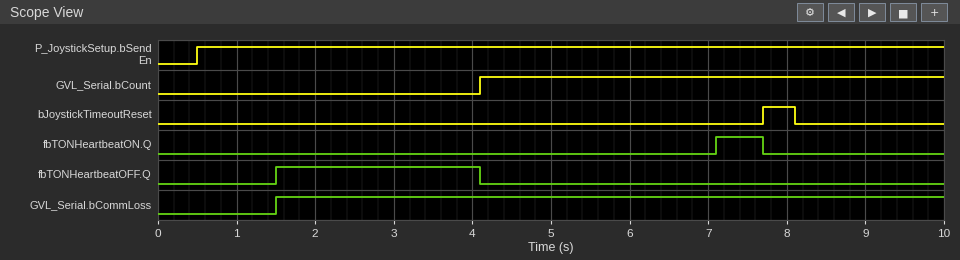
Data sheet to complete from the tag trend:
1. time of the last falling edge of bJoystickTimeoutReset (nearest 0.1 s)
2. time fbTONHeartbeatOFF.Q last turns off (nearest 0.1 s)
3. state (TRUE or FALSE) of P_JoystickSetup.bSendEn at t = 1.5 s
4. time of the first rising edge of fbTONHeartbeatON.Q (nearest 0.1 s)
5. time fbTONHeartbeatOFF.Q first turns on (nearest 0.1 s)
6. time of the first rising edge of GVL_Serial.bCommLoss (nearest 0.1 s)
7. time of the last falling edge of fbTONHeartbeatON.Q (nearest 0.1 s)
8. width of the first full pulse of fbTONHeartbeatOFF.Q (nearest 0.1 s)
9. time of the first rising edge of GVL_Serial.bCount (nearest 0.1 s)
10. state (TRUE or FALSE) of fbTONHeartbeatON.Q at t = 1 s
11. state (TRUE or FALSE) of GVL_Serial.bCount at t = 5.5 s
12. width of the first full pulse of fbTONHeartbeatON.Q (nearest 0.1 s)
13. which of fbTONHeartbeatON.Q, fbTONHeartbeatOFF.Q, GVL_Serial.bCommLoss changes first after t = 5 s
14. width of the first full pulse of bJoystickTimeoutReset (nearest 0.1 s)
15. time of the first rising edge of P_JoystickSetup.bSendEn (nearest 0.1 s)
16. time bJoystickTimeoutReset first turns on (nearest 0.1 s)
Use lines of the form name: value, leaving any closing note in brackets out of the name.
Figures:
time of the last falling edge of bJoystickTimeoutReset: 8.1 s
time fbTONHeartbeatOFF.Q last turns off: 4.1 s
state (TRUE or FALSE) of P_JoystickSetup.bSendEn at t = 1.5 s: TRUE
time of the first rising edge of fbTONHeartbeatON.Q: 7.1 s
time fbTONHeartbeatOFF.Q first turns on: 1.5 s
time of the first rising edge of GVL_Serial.bCommLoss: 1.5 s
time of the last falling edge of fbTONHeartbeatON.Q: 7.7 s
width of the first full pulse of fbTONHeartbeatOFF.Q: 2.6 s
time of the first rising edge of GVL_Serial.bCount: 4.1 s
state (TRUE or FALSE) of fbTONHeartbeatON.Q at t = 1 s: FALSE
state (TRUE or FALSE) of GVL_Serial.bCount at t = 5.5 s: TRUE
width of the first full pulse of fbTONHeartbeatON.Q: 0.6 s
which of fbTONHeartbeatON.Q, fbTONHeartbeatOFF.Q, GVL_Serial.bCommLoss changes first after t = 5 s: fbTONHeartbeatON.Q
width of the first full pulse of bJoystickTimeoutReset: 0.4 s
time of the first rising edge of P_JoystickSetup.bSendEn: 0.5 s
time bJoystickTimeoutReset first turns on: 7.7 s
